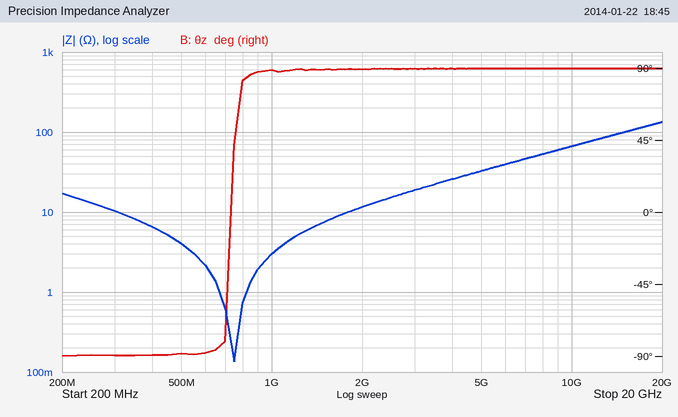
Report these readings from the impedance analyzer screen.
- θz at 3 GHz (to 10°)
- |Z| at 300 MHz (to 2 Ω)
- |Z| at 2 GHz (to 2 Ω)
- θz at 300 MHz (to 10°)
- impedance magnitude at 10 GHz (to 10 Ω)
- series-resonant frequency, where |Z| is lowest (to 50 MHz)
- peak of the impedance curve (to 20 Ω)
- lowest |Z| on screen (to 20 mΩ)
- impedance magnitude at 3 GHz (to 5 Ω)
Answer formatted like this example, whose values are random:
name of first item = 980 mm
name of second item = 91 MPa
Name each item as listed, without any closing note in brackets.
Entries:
θz at 3 GHz = 90°
|Z| at 300 MHz = 10 Ω
|Z| at 2 GHz = 12 Ω
θz at 300 MHz = -90°
impedance magnitude at 10 GHz = 70 Ω
series-resonant frequency, where |Z| is lowest = 750 MHz
peak of the impedance curve = 140 Ω
lowest |Z| on screen = 140 mΩ
impedance magnitude at 3 GHz = 20 Ω
